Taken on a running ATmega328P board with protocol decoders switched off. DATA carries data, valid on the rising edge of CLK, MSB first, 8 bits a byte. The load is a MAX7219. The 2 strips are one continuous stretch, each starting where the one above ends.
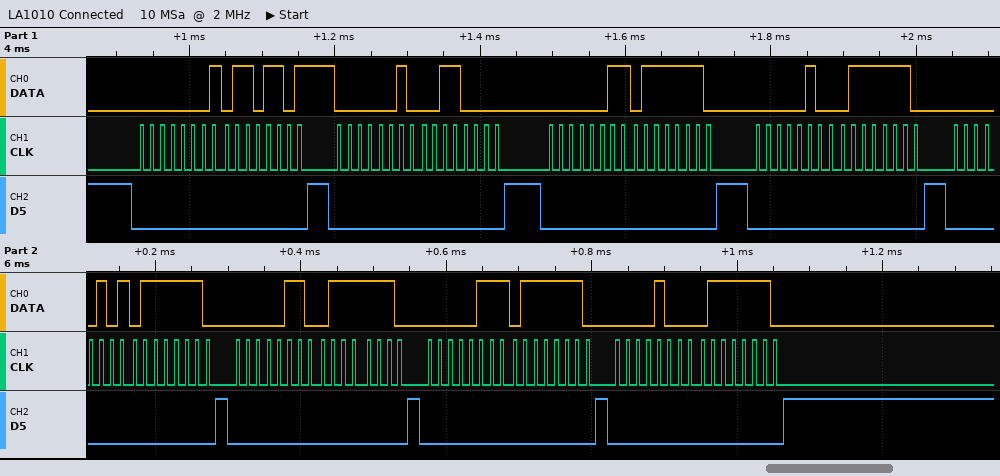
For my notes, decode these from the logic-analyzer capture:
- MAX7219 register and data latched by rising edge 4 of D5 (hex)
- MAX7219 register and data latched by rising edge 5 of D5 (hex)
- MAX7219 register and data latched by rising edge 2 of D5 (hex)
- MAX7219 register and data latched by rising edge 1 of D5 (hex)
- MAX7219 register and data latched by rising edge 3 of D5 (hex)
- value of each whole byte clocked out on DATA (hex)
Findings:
register 0x4, data 0x7E
register 0x5, data 0x7E
register 0x2, data 0x30
register 0x1, data 0x6D
register 0x3, data 0x7E
01 6D 02 30 03 7E 04 7E 05 7E 06 7E 07 7E 08 7E
